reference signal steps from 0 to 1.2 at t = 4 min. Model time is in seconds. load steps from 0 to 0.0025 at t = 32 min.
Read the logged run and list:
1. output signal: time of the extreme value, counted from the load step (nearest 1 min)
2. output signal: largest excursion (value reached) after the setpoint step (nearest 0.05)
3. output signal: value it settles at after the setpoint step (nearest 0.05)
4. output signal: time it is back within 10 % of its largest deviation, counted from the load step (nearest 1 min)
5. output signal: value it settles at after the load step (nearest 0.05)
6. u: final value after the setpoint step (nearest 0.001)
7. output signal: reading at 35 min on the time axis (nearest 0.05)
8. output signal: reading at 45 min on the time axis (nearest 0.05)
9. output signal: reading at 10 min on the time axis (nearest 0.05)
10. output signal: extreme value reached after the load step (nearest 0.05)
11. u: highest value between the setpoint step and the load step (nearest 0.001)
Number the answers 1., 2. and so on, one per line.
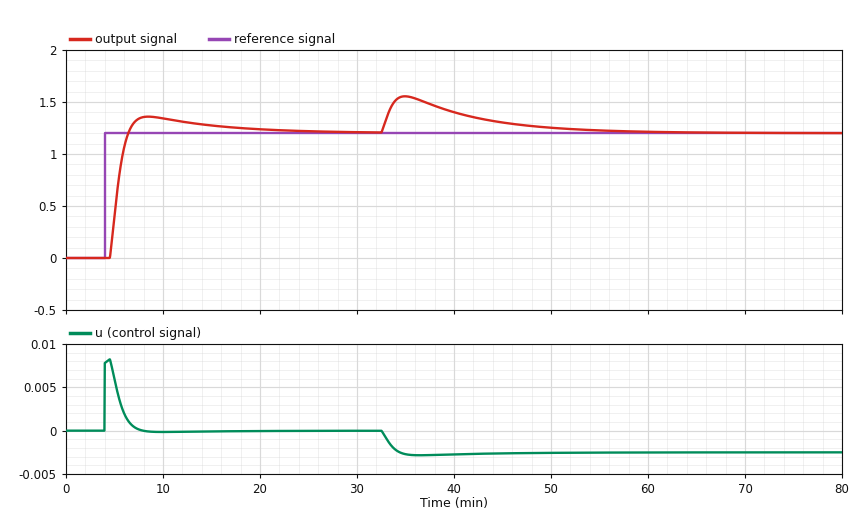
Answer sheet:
1. 3 min
2. 1.35
3. 1.20
4. 21 min
5. 1.20
6. 0.000
7. 1.55
8. 1.30
9. 1.35
10. 1.55
11. 0.008
